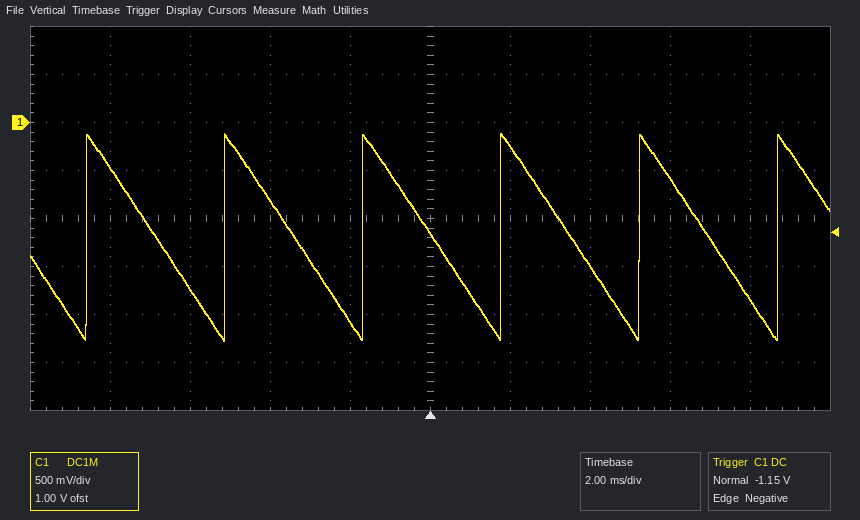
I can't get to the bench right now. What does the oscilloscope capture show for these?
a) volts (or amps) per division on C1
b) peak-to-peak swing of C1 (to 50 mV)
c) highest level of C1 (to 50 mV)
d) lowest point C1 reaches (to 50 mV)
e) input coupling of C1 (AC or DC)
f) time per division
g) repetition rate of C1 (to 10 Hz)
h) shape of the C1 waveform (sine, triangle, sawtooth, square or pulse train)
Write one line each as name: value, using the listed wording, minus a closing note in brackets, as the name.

volts (or amps) per division on C1: 500 mV
peak-to-peak swing of C1: 2.15 V
highest level of C1: -100 mV
lowest point C1 reaches: -2.25 V
input coupling of C1: DC
time per division: 2 ms
repetition rate of C1: 290 Hz
shape of the C1 waveform: sawtooth
